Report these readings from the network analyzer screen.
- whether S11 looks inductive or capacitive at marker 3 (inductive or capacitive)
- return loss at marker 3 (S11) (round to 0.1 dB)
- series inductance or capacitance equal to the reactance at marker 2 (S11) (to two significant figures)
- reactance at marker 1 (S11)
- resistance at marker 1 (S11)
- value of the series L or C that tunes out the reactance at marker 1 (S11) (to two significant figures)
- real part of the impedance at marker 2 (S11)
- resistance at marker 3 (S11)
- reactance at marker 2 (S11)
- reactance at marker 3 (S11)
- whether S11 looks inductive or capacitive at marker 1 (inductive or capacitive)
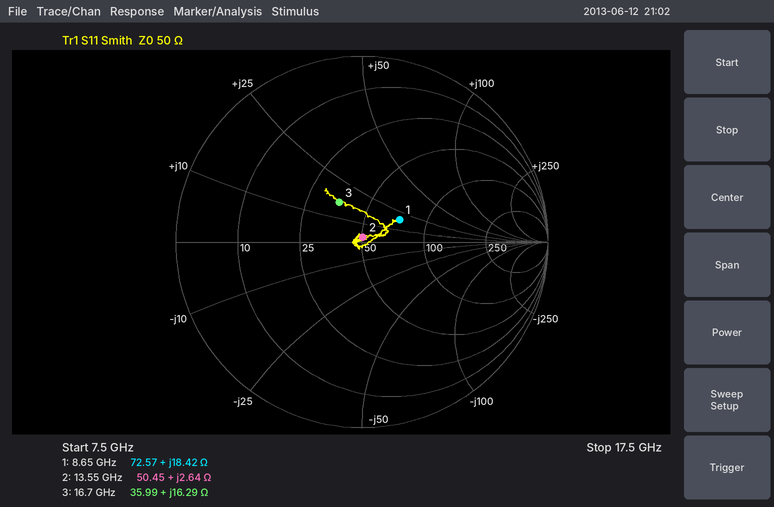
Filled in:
inductive
12.2 dB
31 pH
+18.42 Ω
72.57 Ω
1.00 pF
50.45 Ω
35.99 Ω
+2.64 Ω
+16.29 Ω
inductive
